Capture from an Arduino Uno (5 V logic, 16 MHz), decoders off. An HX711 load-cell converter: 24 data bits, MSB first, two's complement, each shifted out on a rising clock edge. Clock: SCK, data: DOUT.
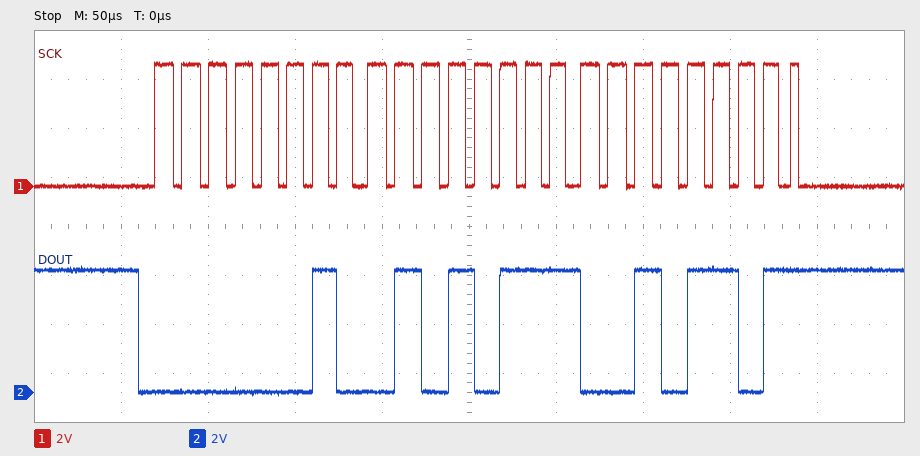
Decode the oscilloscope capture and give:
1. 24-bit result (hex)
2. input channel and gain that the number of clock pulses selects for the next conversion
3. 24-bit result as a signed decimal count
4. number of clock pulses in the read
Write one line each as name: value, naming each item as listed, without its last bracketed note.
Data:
24-bit result: 0x02572D
input channel and gain that the number of clock pulses selects for the next conversion: channel A, gain 128
24-bit result as a signed decimal count: 153389
number of clock pulses in the read: 25
